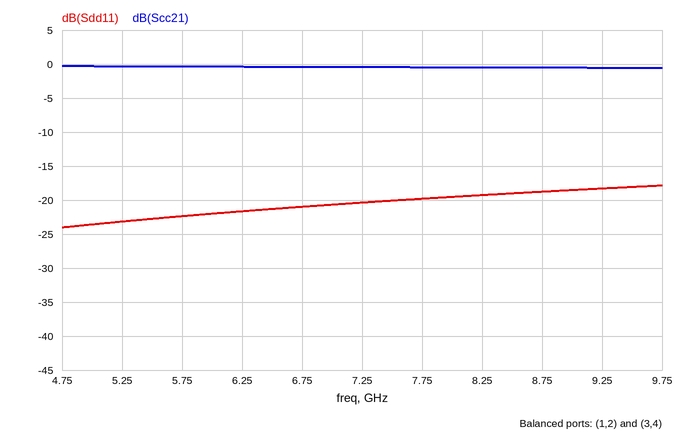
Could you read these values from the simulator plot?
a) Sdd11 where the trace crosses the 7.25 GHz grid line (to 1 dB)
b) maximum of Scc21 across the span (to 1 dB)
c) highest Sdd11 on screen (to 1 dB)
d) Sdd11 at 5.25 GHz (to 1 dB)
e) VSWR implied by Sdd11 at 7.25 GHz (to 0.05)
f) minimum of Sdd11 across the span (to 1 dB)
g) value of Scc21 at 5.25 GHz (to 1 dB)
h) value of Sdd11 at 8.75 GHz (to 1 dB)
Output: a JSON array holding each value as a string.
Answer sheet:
["-20 dB", "0 dB", "-18 dB", "-23 dB", "1.20", "-24 dB", "0 dB", "-19 dB"]
